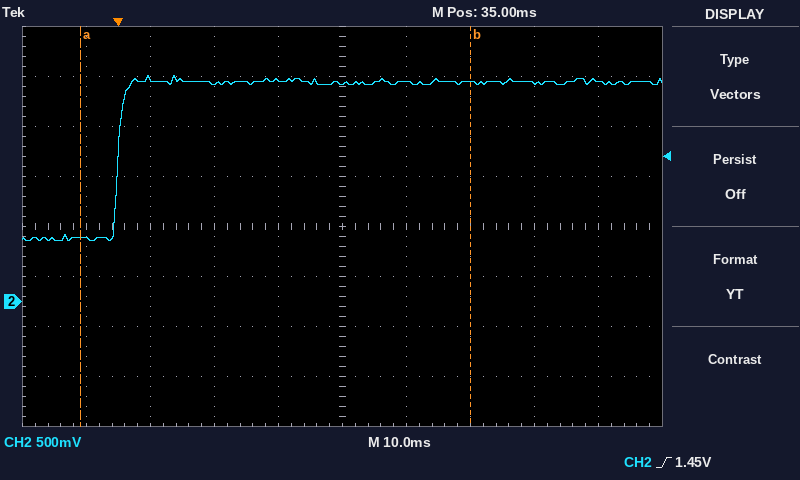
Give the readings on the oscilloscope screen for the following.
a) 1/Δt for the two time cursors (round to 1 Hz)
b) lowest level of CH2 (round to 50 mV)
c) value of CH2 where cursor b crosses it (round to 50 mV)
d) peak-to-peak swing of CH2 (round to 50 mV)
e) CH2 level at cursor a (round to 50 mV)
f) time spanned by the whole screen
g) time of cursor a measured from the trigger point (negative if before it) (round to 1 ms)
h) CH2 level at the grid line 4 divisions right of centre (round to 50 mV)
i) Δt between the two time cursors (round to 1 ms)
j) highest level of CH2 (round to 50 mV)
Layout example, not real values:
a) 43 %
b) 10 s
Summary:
a) 16 Hz
b) 600 mV
c) 2.20 V
d) 1.65 V
e) 650 mV
f) 100 ms
g) -6 ms
h) 2.20 V
i) 61 ms
j) 2.25 V
